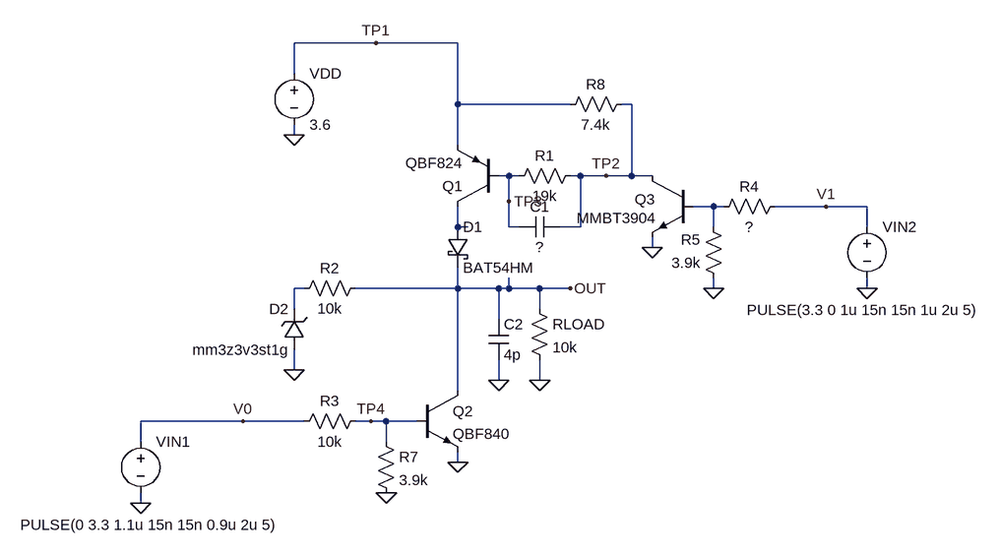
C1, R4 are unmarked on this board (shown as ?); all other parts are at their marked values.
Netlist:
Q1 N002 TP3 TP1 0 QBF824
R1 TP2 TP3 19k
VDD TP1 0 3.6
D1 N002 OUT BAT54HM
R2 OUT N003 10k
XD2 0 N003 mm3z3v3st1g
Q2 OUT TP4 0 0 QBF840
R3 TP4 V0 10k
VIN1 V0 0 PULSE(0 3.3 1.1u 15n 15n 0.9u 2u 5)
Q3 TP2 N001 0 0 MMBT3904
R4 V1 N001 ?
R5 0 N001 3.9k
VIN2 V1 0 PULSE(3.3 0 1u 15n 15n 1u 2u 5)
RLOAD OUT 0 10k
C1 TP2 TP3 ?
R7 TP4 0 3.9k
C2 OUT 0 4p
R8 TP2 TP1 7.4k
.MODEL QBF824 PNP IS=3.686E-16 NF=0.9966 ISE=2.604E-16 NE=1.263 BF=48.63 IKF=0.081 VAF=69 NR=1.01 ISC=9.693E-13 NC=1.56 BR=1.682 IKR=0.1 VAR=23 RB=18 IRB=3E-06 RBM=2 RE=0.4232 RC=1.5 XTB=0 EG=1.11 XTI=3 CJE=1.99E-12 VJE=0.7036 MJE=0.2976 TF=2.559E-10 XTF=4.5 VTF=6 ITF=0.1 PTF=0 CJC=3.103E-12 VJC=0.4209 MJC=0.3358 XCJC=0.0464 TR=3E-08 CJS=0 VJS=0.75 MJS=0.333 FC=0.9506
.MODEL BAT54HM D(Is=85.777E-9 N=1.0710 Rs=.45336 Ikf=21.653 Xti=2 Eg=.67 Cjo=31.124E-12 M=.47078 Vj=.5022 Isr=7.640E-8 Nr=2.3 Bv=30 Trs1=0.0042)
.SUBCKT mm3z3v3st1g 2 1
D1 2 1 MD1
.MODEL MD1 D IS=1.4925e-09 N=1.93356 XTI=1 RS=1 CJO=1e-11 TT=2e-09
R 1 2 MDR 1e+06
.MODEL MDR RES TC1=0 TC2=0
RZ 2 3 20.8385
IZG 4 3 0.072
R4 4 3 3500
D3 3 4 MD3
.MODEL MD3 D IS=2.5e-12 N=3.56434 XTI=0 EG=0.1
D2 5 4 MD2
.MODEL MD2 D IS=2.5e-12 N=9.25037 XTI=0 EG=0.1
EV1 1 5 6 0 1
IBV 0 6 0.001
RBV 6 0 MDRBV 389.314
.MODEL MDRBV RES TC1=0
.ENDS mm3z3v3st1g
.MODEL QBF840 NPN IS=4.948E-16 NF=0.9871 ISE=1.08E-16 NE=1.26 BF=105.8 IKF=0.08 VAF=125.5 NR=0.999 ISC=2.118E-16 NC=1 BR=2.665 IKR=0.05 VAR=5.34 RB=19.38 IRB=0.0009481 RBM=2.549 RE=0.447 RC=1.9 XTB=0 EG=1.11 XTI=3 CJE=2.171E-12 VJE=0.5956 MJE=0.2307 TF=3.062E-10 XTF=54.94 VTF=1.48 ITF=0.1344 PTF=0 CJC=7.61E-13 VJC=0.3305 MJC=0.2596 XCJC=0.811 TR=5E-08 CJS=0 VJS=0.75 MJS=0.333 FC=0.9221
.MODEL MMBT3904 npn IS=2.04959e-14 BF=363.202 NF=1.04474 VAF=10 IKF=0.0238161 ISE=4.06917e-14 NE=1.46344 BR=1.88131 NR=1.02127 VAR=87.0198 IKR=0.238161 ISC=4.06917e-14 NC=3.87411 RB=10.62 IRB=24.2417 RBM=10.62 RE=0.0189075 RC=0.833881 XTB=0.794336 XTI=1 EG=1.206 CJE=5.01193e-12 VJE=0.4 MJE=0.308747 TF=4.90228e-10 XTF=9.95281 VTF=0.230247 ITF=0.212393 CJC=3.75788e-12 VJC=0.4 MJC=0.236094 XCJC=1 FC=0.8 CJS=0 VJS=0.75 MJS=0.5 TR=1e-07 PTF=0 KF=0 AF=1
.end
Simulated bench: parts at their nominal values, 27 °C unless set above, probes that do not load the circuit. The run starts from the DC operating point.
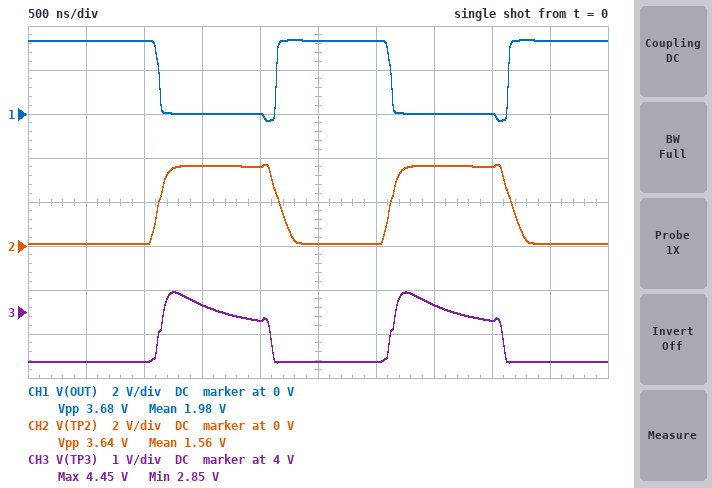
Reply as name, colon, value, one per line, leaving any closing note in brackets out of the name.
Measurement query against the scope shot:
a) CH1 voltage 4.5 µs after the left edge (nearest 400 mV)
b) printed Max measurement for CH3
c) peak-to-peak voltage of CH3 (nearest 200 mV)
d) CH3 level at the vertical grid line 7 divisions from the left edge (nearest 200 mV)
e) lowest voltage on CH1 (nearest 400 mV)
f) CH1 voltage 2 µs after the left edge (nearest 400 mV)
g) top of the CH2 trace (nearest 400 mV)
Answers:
CH1 voltage 4.5 µs after the left edge: 3.2 V
printed Max measurement for CH3: 4.45 V
peak-to-peak voltage of CH3: 1.6 V
CH3 level at the vertical grid line 7 divisions from the left edge: 4.2 V
lowest voltage on CH1: -400 mV
CH1 voltage 2 µs after the left edge: 0 V
top of the CH2 trace: 3.6 V
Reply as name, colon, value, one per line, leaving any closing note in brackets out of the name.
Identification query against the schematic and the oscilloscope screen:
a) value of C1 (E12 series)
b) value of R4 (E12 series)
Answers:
value of C1: 22 pF
value of R4: 12 kΩ
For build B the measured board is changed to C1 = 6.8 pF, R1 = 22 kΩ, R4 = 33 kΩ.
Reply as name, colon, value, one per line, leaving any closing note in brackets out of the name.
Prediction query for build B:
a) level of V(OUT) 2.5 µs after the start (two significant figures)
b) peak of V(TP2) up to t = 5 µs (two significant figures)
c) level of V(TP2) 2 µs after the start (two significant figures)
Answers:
level of V(OUT) 2.5 µs after the start: -17 mV
peak of V(TP2) up to t = 5 µs: 3.6 V
level of V(TP2) 2 µs after the start: 3.6 V
